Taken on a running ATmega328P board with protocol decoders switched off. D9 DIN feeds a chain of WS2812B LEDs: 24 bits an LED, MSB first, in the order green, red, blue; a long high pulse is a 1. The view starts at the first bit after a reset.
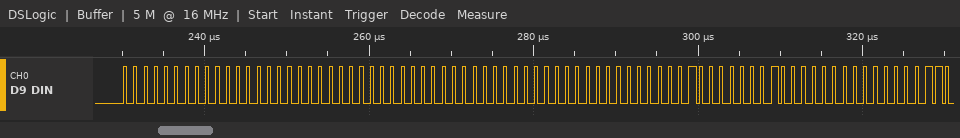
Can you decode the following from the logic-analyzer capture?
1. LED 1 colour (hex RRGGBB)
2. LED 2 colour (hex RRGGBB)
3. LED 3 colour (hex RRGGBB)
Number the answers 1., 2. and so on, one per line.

1. #000000
2. #000000
3. #010100
